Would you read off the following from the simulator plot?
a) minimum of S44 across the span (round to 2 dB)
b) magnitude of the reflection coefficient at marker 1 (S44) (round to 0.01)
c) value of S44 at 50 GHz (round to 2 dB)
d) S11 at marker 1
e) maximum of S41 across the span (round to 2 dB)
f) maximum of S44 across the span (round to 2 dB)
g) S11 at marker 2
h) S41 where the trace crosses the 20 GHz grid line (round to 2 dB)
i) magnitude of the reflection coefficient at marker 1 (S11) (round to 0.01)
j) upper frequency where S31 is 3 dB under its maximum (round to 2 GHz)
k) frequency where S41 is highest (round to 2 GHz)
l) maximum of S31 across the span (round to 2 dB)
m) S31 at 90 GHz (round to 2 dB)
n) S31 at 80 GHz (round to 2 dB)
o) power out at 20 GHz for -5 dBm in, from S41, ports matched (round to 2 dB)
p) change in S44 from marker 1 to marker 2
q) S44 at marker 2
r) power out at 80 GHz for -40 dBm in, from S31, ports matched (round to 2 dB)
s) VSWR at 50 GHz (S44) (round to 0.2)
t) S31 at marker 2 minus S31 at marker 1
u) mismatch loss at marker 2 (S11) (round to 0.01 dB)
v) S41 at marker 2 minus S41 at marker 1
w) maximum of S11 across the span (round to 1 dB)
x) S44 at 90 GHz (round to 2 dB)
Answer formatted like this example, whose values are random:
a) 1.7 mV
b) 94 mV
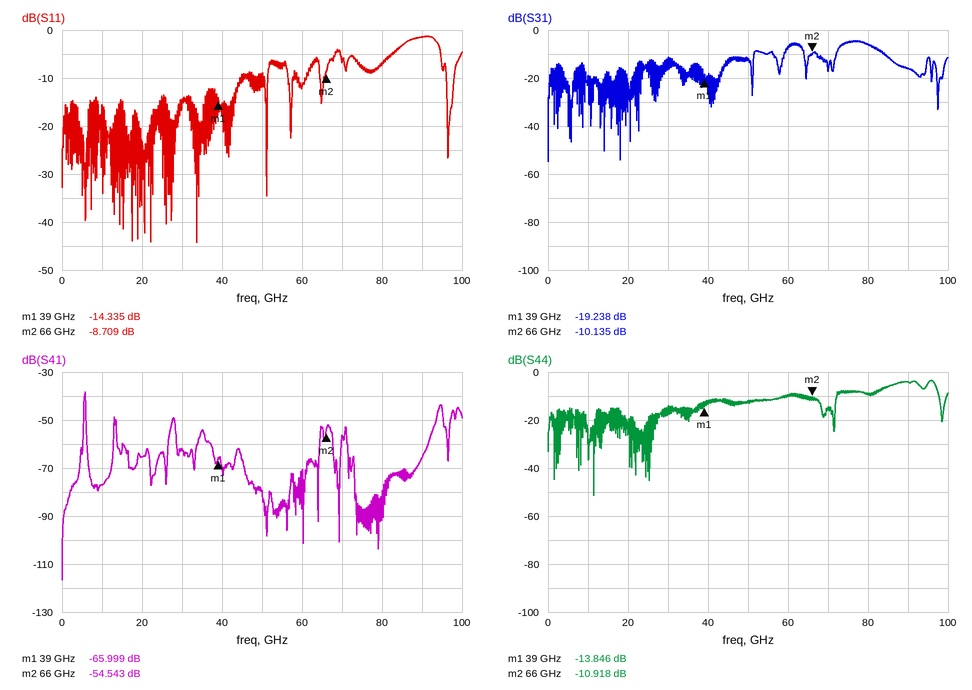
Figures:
a) -52 dB
b) 0.20
c) -12 dB
d) -14.335 dB
e) -38 dB
f) -4 dB
g) -8.709 dB
h) -66 dB
i) 0.19
j) 82 GHz
k) 6 GHz
l) -4 dB
m) -16 dB
n) -6 dB
o) -70 dBm
p) 2.928 dB
q) -10.918 dB
r) -46 dBm
s) 1.6
t) 9.103 dB
u) 0.63 dB
v) 11.456 dB
w) -1 dB
x) -4 dB
